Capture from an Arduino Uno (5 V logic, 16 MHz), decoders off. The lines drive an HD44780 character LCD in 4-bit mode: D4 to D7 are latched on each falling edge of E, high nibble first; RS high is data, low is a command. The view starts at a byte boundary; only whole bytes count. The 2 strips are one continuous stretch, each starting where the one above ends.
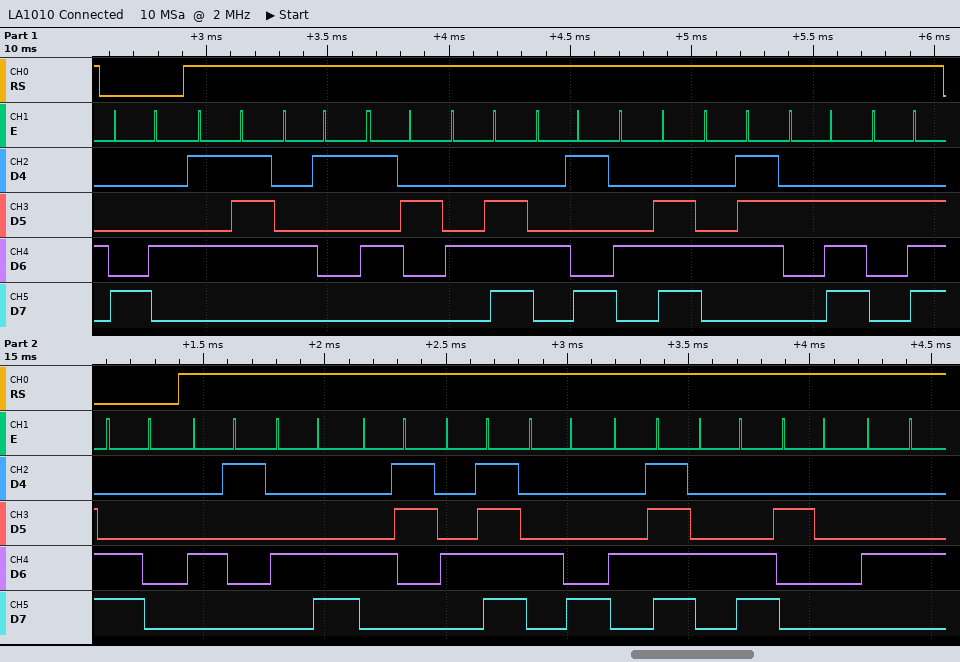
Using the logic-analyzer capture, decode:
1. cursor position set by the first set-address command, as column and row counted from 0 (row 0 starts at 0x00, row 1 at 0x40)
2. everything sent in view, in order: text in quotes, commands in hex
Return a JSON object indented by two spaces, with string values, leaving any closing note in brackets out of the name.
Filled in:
{
  "cursor position set by the first set-address command, as column and row counted from 0": "column 4, row 0",
  "everything sent in view, in order: text in quotes, commands in hex": "0x84 \"WARNING..\" 0xC0 \"ALCOHOL D\""
}
